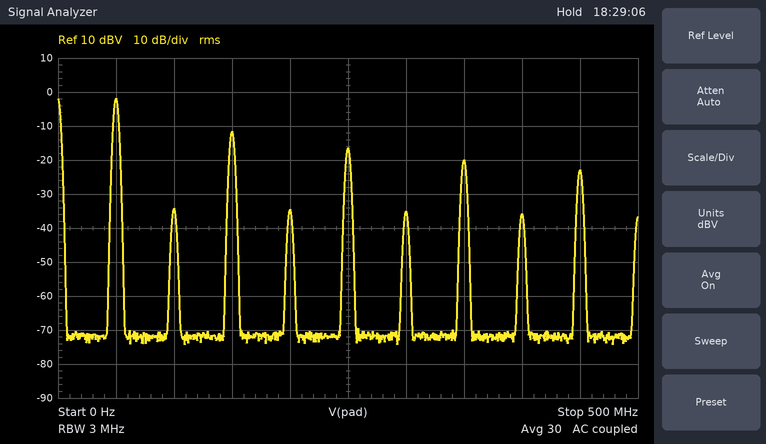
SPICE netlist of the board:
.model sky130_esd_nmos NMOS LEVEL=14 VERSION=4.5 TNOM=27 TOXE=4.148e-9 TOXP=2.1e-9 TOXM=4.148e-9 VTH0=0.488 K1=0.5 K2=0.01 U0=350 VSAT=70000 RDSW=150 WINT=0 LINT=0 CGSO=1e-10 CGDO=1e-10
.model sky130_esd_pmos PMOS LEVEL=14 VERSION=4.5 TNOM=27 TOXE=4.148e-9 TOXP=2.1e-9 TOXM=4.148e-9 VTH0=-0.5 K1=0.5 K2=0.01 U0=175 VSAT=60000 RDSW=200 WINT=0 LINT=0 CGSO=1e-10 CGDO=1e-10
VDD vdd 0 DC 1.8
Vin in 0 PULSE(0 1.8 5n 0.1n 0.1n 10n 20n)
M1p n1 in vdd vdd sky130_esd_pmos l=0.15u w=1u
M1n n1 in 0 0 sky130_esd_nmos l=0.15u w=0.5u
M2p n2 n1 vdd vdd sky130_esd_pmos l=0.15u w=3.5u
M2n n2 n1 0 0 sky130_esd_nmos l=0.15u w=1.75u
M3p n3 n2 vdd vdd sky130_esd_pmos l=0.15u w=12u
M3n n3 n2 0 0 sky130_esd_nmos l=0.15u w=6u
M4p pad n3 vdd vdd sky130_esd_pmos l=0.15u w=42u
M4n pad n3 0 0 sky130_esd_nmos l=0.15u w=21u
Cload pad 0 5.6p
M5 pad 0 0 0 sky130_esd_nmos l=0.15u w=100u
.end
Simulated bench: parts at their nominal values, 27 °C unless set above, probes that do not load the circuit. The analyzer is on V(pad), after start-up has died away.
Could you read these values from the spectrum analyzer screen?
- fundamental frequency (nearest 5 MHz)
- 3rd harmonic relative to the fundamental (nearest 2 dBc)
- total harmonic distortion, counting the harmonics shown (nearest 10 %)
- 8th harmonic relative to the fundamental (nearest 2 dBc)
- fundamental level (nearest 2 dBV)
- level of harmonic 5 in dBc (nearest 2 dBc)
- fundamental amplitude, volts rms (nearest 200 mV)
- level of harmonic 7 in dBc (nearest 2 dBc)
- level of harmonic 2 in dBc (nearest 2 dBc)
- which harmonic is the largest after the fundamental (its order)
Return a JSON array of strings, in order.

["50 MHz", "-10 dBc", "40 %", "-34 dBc", "-2 dBV", "-14 dBc", "800 mV", "-18 dBc", "-32 dBc", "3"]
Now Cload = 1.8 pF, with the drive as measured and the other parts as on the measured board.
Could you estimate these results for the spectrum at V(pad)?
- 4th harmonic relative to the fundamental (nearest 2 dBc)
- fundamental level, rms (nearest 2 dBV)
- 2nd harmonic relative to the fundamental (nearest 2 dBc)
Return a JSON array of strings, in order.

["-34 dBc", "-2 dBV", "-34 dBc"]
